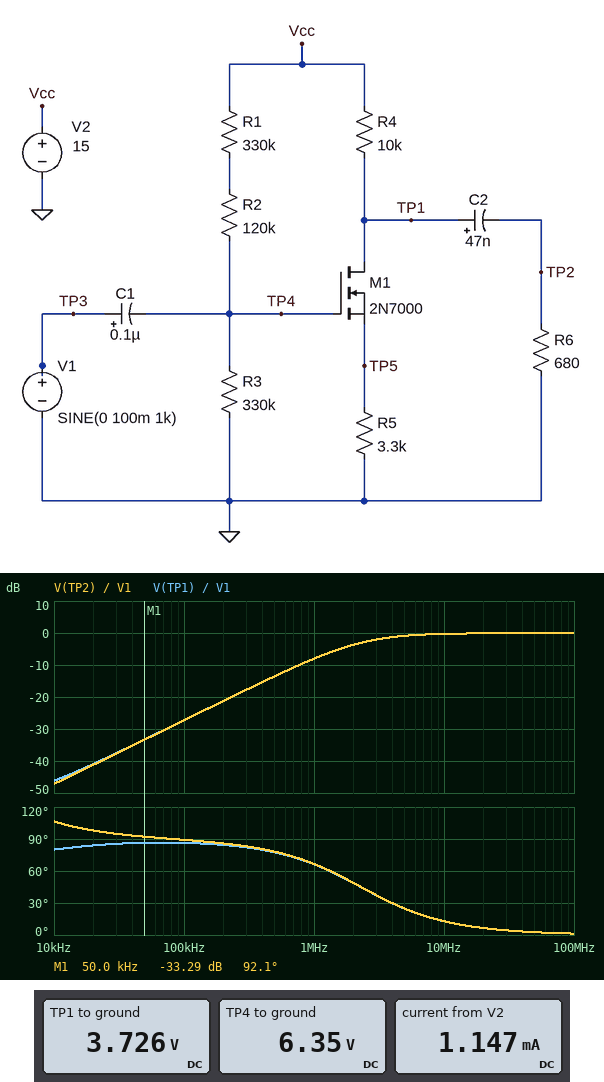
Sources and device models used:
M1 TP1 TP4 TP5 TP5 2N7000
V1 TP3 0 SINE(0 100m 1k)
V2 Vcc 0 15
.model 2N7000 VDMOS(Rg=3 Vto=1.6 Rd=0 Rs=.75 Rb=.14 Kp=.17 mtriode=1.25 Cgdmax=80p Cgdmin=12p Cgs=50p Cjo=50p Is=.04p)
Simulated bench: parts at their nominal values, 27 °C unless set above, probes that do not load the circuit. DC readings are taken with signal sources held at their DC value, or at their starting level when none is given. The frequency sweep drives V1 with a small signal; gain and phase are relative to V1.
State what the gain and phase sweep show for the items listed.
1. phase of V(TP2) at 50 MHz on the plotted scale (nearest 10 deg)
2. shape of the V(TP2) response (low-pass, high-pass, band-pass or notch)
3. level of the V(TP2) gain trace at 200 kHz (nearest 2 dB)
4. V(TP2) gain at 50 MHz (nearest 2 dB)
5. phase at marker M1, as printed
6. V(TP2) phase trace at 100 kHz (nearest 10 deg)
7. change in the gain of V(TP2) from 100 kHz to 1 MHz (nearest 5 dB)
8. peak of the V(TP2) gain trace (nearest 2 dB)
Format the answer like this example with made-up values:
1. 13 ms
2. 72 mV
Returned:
1. 0 deg
2. high-pass
3. -22 dB
4. 0 dB
5. 92.1 deg
6. 90 deg
7. 20 dB
8. 0 dB
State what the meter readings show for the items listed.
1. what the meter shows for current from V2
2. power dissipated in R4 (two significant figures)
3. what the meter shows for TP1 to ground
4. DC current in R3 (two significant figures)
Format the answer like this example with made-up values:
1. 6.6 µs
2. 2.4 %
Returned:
1. 1.147 mA
2. 13 mW
3. 3.726 V
4. 19 µA
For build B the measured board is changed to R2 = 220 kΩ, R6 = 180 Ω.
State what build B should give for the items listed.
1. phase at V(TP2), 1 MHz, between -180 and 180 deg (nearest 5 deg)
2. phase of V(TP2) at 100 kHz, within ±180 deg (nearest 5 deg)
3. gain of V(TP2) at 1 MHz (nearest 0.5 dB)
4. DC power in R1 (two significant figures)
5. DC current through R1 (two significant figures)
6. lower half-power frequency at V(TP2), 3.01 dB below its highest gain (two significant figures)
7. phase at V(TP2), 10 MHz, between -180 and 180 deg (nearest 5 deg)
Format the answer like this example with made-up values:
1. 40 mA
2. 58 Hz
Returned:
1. 85 deg
2. 100 deg
3. -17.5 dB
4. 96 µW
5. 17 µA
6. 7.5 MHz
7. 35 deg
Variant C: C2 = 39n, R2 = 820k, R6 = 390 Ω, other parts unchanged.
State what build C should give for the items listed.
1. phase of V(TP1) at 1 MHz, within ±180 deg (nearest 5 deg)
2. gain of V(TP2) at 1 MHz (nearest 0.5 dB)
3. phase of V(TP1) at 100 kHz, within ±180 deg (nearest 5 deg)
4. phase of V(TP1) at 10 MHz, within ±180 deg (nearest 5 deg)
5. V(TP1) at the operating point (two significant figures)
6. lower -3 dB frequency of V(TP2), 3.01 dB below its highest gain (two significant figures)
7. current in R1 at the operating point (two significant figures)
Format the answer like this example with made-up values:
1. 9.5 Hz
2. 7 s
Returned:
1. 155 deg
2. -18.5 dB
3. 170 deg
4. 85 deg
5. 9.8 V
6. 14 MHz
7. 10 µA
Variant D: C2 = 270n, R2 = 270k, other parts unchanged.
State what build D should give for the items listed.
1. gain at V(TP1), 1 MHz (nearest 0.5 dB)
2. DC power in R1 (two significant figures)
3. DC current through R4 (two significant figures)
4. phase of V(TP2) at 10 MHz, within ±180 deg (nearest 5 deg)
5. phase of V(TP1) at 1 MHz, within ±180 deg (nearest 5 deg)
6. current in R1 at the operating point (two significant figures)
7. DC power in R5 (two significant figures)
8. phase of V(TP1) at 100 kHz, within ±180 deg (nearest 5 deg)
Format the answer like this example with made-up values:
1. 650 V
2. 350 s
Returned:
1. -9.0 dB
2. 86 µW
3. 1.1 mA
4. 20 deg
5. 105 deg
6. 16 µA
7. 4.0 mW
8. 170 deg
